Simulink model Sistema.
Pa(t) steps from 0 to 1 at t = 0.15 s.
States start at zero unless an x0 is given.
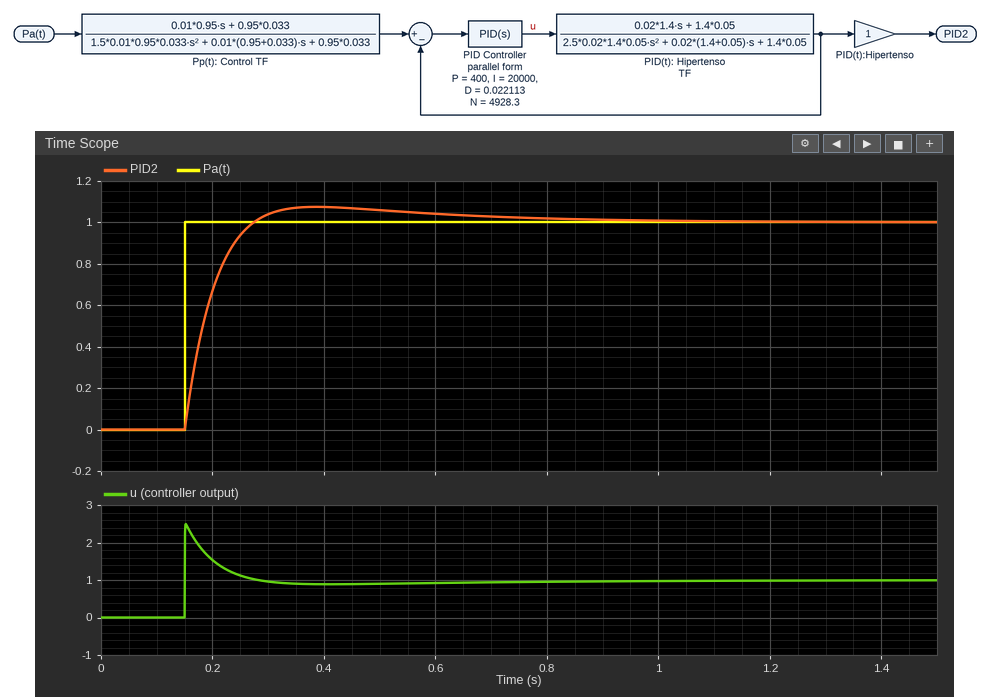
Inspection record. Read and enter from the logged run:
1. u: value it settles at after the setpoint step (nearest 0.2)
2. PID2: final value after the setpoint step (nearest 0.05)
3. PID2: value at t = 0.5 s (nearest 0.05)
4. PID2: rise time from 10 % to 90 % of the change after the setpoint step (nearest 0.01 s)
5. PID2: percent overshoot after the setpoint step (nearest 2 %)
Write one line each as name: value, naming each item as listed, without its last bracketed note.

u: value it settles at after the setpoint step: 1.0
PID2: final value after the setpoint step: 1.00
PID2: value at t = 0.5 s: 1.05
PID2: rise time from 10 % to 90 % of the change after the setpoint step: 0.08 s
PID2: percent overshoot after the setpoint step: 8 %
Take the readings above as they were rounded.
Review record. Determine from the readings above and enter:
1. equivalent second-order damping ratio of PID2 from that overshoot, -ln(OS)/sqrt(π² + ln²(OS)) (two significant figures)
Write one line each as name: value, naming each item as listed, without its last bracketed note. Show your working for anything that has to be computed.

equivalent second-order damping ratio of PID2 from that overshoot, -ln(OS)/sqrt(π² + ln²(OS)): ln(0.08) = -2.526; 2.526 / sqrt(9.870 + 6.379) = 0.63
